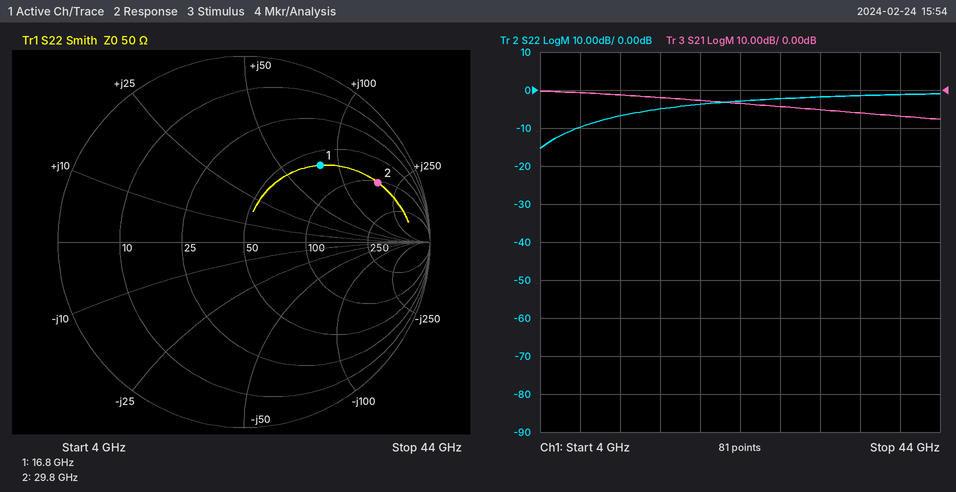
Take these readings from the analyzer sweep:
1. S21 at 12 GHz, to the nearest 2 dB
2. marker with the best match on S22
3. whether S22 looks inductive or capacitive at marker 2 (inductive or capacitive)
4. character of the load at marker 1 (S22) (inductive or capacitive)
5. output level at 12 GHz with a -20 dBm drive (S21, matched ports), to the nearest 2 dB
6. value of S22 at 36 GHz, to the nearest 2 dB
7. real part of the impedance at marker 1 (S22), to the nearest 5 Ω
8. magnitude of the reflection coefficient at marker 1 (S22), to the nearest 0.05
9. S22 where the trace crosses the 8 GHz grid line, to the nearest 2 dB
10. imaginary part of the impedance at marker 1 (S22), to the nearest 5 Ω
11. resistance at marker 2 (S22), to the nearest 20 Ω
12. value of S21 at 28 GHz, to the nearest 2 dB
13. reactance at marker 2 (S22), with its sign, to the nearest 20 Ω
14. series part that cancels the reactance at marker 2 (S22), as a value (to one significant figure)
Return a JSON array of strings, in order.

["-2 dB", "marker 1", "inductive", "inductive", "-22 dBm", "-2 dB", "65 Ω", "0.60", "-10 dB", "+80 Ω", "100 Ω", "-4 dB", "+180 Ω", "30 fF"]
